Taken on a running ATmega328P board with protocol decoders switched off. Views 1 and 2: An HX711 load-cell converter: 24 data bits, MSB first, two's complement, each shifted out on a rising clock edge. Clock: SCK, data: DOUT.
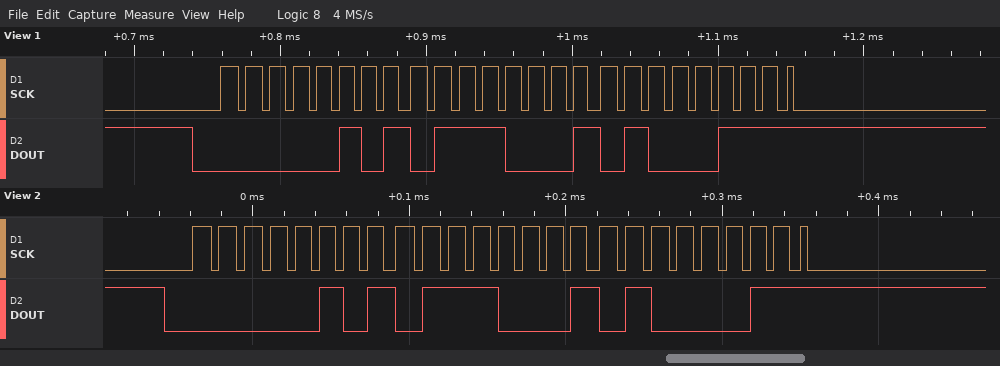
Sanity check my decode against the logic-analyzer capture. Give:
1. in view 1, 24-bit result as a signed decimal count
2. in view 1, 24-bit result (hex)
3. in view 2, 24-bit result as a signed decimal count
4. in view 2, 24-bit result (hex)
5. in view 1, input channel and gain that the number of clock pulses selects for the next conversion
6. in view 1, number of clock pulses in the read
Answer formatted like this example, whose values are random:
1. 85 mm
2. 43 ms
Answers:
1. 356679
2. 0x057147
3. 356675
4. 0x057143
5. channel A, gain 128
6. 25
